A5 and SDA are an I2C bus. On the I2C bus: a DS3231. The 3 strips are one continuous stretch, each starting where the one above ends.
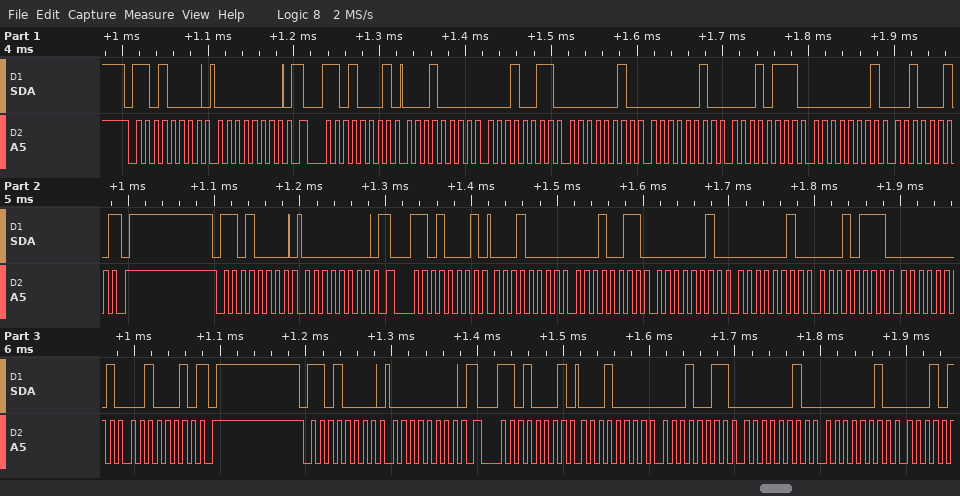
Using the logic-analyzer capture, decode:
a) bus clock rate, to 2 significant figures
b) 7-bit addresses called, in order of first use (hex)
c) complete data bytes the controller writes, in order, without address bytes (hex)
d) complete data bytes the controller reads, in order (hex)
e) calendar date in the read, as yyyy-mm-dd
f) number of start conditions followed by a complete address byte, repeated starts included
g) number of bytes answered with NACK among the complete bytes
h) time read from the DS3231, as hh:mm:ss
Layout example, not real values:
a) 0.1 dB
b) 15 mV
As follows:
a) 100 kHz
b) 0x68
c) 00 00 00
d) 10 13 02 02 17 01 22 10 13 02 02 17 01 22 10 13 02 02
e) 2022-01-17
f) 6
g) 2
h) 02:13:10
